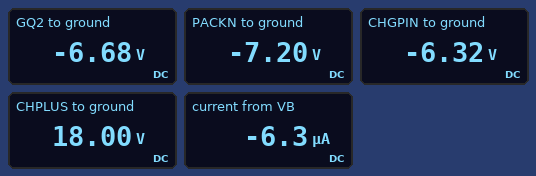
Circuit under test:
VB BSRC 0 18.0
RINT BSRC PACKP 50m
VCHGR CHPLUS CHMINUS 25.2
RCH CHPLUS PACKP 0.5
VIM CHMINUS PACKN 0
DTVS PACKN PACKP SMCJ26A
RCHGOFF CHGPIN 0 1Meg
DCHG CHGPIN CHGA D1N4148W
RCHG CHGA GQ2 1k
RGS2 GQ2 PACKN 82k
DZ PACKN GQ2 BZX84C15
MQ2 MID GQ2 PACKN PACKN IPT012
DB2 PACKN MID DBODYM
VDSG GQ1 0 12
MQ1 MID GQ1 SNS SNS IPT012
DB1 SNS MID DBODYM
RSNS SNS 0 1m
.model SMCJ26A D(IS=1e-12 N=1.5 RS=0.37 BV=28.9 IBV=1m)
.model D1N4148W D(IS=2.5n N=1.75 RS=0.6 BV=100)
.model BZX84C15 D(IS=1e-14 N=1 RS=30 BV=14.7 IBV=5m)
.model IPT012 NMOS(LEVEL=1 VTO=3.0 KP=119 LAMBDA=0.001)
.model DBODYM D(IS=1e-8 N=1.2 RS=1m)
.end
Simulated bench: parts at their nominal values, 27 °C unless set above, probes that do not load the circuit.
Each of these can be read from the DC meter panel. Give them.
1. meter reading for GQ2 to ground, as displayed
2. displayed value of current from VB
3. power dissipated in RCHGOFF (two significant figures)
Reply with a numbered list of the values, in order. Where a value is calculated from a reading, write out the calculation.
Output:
1. -6.68 V
2. -6.3 µA
3. (0 V - (-6.32 V))^2 / 1 MΩ = 40 µW
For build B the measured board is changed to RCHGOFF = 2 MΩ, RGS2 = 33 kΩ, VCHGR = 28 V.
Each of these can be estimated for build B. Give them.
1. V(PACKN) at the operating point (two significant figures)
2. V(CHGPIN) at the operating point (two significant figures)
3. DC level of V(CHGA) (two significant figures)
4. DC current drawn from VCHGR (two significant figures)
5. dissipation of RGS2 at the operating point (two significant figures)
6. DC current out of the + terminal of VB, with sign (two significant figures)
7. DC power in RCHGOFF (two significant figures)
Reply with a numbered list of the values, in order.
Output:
1. -10 V
2. -9.5 V
3. -9.8 V
4. 4.8 µA
5. 740 nW
6. -4.8 µA
7. 45 µW
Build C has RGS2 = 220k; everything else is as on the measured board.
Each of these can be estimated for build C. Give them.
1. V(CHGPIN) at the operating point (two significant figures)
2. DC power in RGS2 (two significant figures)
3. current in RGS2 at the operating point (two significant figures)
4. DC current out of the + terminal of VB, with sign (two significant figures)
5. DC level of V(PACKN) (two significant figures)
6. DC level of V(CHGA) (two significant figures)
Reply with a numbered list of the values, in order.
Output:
1. -5.6 V
2. 6.9 µW
3. 5.6 µA
4. -5.6 µA
5. -7.2 V
6. -6.0 V
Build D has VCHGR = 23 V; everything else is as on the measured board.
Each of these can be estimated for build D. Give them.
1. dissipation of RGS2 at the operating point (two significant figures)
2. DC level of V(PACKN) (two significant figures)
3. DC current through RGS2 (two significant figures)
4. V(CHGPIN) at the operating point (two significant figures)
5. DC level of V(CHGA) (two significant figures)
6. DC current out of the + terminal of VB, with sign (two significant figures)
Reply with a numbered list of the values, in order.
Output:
1. 1.5 µW
2. -5.0 V
3. 4.3 µA
4. -4.3 V
5. -4.6 V
6. -4.3 µA
